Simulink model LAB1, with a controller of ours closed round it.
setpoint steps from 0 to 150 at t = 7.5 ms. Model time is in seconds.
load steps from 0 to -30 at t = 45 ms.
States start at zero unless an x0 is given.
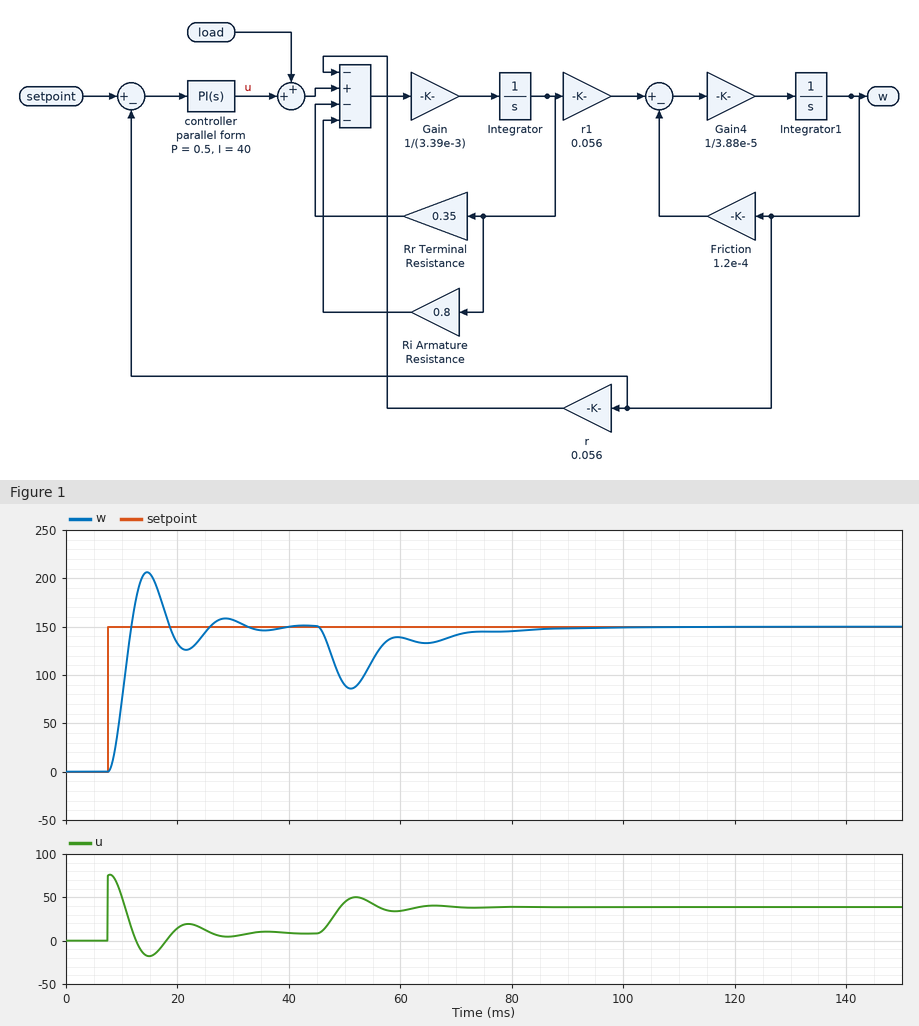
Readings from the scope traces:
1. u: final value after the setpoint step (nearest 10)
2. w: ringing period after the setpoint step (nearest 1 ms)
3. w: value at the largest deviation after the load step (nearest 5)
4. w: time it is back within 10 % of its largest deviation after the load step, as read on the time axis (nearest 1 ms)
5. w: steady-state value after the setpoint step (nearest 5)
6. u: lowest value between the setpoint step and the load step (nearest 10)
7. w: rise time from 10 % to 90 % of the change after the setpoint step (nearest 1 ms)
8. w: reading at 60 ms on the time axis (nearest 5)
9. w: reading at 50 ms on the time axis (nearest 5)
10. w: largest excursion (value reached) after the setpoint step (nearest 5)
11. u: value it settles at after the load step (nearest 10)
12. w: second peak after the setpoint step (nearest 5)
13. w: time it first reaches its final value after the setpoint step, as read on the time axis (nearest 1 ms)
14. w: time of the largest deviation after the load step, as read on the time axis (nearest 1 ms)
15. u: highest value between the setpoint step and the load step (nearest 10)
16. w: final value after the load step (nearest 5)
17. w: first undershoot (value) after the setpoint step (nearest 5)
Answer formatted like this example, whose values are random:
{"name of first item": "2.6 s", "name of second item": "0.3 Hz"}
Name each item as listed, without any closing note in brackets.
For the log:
{"u: final value after the setpoint step": "10", "w: ringing period after the setpoint step": "14 ms", "w: value at the largest deviation after the load step": "85", "w: time it is back within 10 % of its largest deviation after the load step, as read on the time axis": "72 ms", "w: steady-state value after the setpoint step": "150", "u: lowest value between the setpoint step and the load step": "-20", "w: rise time from 10 % to 90 % of the change after the setpoint step": "3 ms", "w: reading at 60 ms on the time axis": "140", "w: reading at 50 ms on the time axis": "90", "w: largest excursion (value reached) after the setpoint step": "205", "u: value it settles at after the load step": "40", "w: second peak after the setpoint step": "160", "w: time it first reaches its final value after the setpoint step, as read on the time axis": "12 ms", "w: time of the largest deviation after the load step, as read on the time axis": "51 ms", "u: highest value between the setpoint step and the load step": "80", "w: final value after the load step": "150", "w: first undershoot (value) after the setpoint step": "125"}
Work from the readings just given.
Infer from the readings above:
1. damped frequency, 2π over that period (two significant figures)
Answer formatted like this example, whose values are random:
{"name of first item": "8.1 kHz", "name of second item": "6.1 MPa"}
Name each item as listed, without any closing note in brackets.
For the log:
{"damped frequency, 2π over that period": "0.45 rad/ms"}
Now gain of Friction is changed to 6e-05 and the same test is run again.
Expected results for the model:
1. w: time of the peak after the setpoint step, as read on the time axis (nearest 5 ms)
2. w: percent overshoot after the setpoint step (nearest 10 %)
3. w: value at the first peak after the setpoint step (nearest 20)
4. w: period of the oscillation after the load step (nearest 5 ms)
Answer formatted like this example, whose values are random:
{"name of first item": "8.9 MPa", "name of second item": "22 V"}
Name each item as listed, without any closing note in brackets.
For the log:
{"w: time of the peak after the setpoint step, as read on the time axis": "15 ms", "w: percent overshoot after the setpoint step": "40 %", "w: value at the first peak after the setpoint step": "200", "w: period of the oscillation after the load step": "15 ms"}
